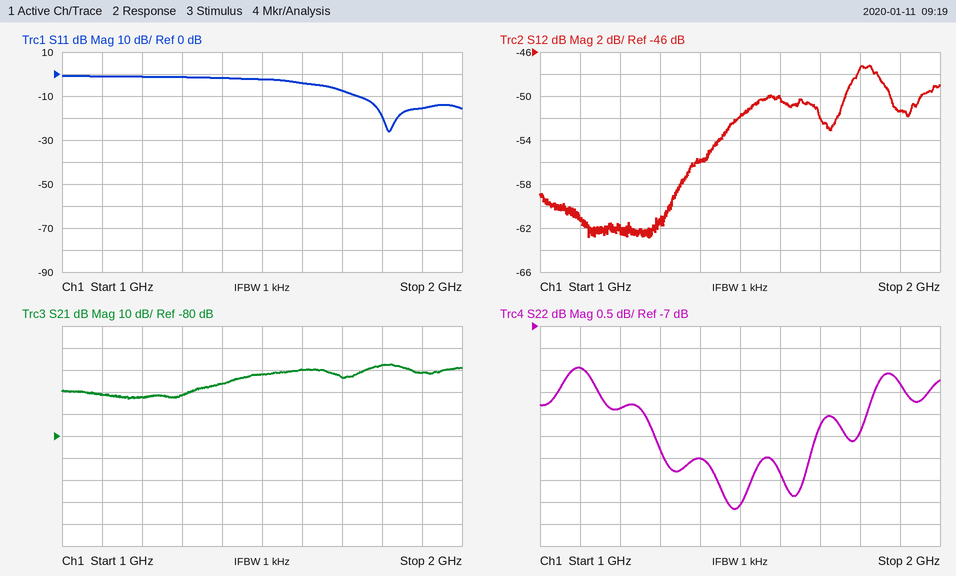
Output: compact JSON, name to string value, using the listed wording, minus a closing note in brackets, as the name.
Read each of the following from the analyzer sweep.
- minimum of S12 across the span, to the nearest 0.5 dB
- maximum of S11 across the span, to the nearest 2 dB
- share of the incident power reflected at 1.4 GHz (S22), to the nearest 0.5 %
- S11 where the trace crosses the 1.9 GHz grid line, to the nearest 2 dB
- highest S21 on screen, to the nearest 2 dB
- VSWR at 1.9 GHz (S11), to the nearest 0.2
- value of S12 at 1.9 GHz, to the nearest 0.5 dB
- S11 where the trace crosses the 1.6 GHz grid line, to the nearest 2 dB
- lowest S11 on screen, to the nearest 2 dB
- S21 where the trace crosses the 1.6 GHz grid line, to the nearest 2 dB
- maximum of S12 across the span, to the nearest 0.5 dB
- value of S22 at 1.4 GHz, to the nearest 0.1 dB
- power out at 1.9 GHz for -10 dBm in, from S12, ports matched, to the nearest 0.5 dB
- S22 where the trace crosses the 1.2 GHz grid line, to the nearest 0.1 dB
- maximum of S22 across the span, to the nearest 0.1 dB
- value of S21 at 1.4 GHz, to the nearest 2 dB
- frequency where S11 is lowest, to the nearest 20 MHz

{"minimum of S12 across the span, to the nearest 0.5 dB": "-63.0 dB", "maximum of S11 across the span, to the nearest 2 dB": "0 dB", "share of the incident power reflected at 1.4 GHz (S22), to the nearest 0.5 %": "10.0 %", "S11 where the trace crosses the 1.9 GHz grid line, to the nearest 2 dB": "-16 dB", "highest S21 on screen, to the nearest 2 dB": "-48 dB", "VSWR at 1.9 GHz (S11), to the nearest 0.2": "1.4", "value of S12 at 1.9 GHz, to the nearest 0.5 dB": "-51.5 dB", "S11 where the trace crosses the 1.6 GHz grid line, to the nearest 2 dB": "-4 dB", "lowest S11 on screen, to the nearest 2 dB": "-26 dB", "S21 where the trace crosses the 1.6 GHz grid line, to the nearest 2 dB": "-50 dB", "maximum of S12 across the span, to the nearest 0.5 dB": "-47.0 dB", "value of S22 at 1.4 GHz, to the nearest 0.1 dB": "-10.0 dB", "power out at 1.9 GHz for -10 dBm in, from S12, ports matched, to the nearest 0.5 dB": "-61.5 dBm", "S22 where the trace crosses the 1.2 GHz grid line, to the nearest 0.1 dB": "-8.9 dB", "maximum of S22 across the span, to the nearest 0.1 dB": "-7.9 dB", "value of S21 at 1.4 GHz, to the nearest 2 dB": "-56 dB", "frequency where S11 is lowest, to the nearest 20 MHz": "1.82 GHz"}
